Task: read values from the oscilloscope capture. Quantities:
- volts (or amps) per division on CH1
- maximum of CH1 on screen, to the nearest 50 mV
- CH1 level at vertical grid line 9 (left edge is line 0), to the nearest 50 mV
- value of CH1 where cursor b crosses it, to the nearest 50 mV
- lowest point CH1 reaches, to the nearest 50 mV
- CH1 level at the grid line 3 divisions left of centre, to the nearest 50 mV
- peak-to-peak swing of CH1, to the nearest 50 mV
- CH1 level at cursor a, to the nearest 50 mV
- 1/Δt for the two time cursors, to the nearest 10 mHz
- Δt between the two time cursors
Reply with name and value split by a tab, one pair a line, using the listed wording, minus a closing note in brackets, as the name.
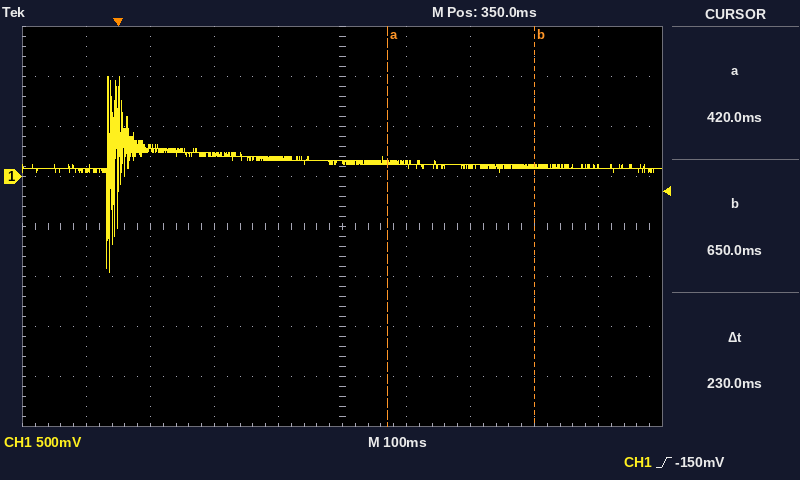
volts (or amps) per division on CH1	500 mV
maximum of CH1 on screen, to the nearest 50 mV	1.00 V
CH1 level at vertical grid line 9 (left edge is line 0), to the nearest 50 mV	100 mV
value of CH1 where cursor b crosses it, to the nearest 50 mV	100 mV
lowest point CH1 reaches, to the nearest 50 mV	-950 mV
CH1 level at the grid line 3 divisions left of centre, to the nearest 50 mV	300 mV
peak-to-peak swing of CH1, to the nearest 50 mV	1.95 V
CH1 level at cursor a, to the nearest 50 mV	150 mV
1/Δt for the two time cursors, to the nearest 10 mHz	4.35 Hz
Δt between the two time cursors	230 ms
